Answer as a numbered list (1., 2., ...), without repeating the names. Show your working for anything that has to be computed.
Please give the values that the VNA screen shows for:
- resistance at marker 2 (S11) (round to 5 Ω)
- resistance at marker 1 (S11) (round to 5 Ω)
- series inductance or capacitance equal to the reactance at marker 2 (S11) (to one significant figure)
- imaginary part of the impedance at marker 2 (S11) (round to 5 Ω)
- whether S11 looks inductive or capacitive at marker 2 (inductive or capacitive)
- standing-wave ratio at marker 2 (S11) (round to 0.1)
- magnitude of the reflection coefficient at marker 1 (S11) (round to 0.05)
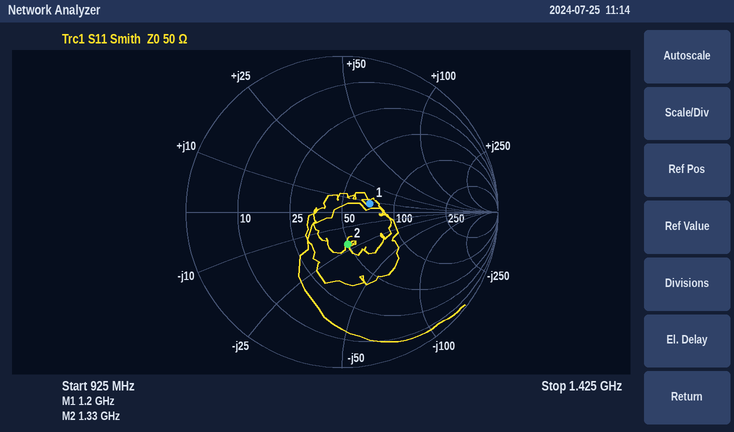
1. 50 Ω
2. 70 Ω
3. C = 1/(2π × 1.33 GHz × 20 Ω) ≈ 6 pF
4. -20 Ω
5. capacitive
6. 1.5
7. 0.20
